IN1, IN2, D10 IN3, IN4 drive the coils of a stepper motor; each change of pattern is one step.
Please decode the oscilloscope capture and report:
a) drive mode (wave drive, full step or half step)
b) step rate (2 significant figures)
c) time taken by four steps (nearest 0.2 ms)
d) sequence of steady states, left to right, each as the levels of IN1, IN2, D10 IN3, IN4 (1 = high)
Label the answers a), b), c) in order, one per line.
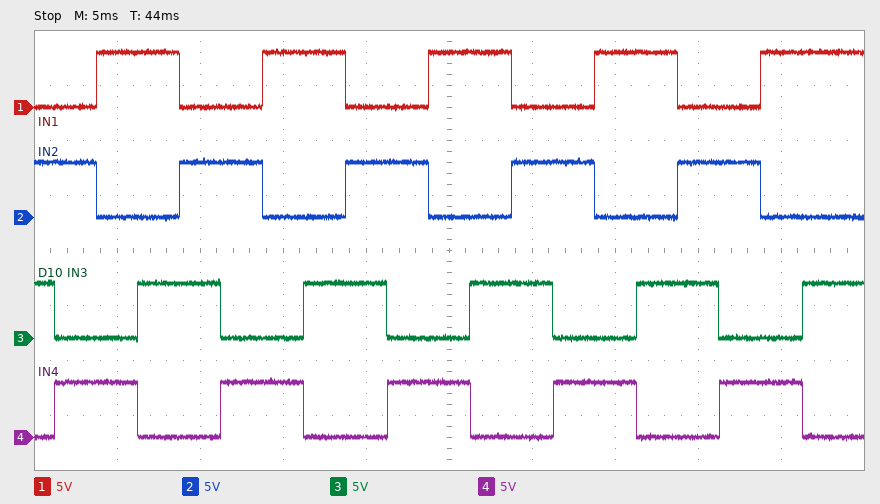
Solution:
a) full step
b) 400 steps/s
c) 10.0 ms
d) 0110 0101 1001 1010 0110 0101 1001 1010 0110 0101 1001 1010 0110 0101 1001 1010 0110 0101 1001 1010
